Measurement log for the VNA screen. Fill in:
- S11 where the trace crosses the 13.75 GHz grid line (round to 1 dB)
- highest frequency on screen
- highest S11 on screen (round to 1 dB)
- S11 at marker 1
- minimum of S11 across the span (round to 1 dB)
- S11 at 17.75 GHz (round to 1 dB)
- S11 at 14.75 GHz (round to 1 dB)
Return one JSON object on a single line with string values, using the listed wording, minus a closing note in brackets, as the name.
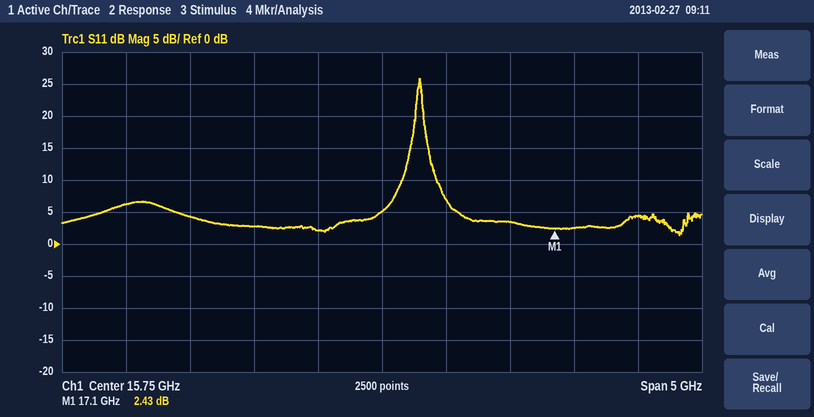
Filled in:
{"S11 where the trace crosses the 13.75 GHz grid line": "6 dB", "highest frequency on screen": "18.25 GHz", "highest S11 on screen": "26 dB", "S11 at marker 1": "2.43 dB", "minimum of S11 across the span": "1 dB", "S11 at 17.75 GHz": "4 dB", "S11 at 14.75 GHz": "3 dB"}
